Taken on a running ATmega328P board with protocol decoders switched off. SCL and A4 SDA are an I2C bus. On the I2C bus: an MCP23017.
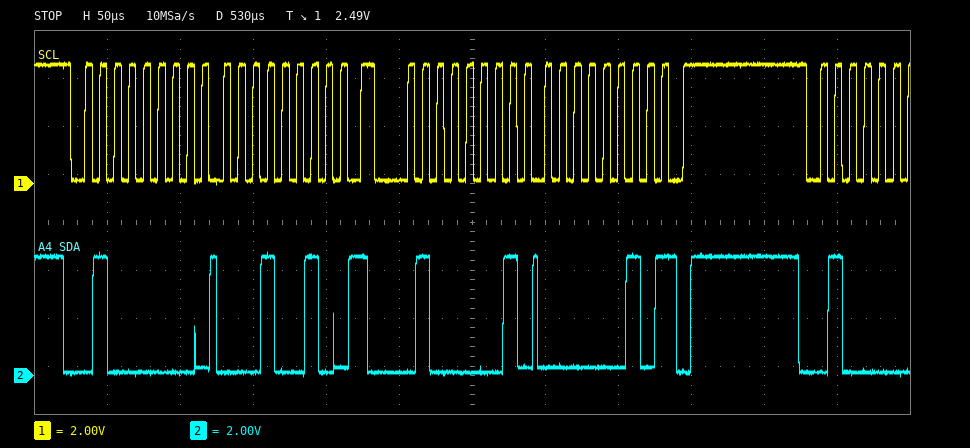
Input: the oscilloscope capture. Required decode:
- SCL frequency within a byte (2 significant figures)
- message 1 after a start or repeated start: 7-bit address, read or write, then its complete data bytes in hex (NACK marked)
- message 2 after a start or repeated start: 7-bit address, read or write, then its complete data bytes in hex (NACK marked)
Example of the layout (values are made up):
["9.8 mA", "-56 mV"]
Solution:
["100 kHz", "0x20 write: 12", "0x20 read: 02 NACK"]
